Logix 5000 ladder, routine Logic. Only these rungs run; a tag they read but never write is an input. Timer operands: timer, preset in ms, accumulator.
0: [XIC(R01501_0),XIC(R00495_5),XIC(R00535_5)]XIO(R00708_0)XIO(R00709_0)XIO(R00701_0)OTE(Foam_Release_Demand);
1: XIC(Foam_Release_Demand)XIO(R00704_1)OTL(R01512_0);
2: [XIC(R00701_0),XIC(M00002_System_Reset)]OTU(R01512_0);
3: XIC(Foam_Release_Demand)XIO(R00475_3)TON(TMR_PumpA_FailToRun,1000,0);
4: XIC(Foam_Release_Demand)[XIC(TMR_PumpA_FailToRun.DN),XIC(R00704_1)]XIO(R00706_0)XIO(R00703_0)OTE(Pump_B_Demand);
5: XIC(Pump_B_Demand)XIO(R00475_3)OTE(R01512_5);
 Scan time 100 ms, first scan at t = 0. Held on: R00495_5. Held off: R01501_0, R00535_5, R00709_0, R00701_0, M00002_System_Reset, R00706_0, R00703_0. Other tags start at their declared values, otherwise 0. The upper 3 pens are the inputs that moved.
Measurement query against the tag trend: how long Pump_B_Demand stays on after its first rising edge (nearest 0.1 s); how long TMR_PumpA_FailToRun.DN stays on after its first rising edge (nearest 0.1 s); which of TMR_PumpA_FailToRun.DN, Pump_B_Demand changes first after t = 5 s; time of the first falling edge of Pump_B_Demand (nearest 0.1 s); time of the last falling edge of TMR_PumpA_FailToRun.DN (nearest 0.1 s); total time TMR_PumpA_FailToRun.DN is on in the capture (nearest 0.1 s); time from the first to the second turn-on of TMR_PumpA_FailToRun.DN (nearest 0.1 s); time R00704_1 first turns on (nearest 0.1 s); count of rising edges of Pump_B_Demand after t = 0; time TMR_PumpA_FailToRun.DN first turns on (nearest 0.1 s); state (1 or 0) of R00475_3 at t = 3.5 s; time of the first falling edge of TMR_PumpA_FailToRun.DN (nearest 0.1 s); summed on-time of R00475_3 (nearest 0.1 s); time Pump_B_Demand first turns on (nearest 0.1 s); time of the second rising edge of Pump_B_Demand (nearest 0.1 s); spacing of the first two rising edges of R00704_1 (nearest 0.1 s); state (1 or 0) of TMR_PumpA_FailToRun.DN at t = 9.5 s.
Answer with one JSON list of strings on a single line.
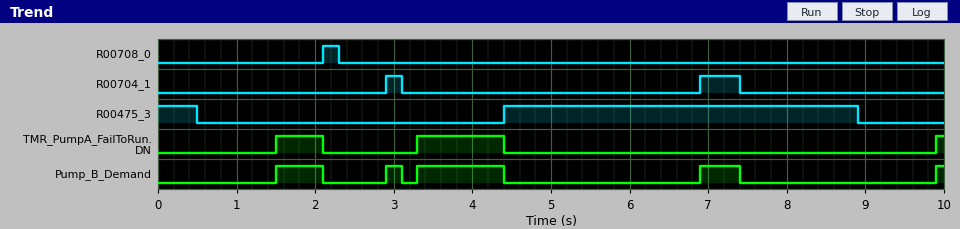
["0.6 s", "0.6 s", "Pump_B_Demand", "2.1 s", "4.4 s", "1.8 s", "1.8 s", "2.9 s", "5", "1.5 s", "0", "2.1 s", "5.0 s", "1.5 s", "2.9 s", "4.0 s", "0"]
